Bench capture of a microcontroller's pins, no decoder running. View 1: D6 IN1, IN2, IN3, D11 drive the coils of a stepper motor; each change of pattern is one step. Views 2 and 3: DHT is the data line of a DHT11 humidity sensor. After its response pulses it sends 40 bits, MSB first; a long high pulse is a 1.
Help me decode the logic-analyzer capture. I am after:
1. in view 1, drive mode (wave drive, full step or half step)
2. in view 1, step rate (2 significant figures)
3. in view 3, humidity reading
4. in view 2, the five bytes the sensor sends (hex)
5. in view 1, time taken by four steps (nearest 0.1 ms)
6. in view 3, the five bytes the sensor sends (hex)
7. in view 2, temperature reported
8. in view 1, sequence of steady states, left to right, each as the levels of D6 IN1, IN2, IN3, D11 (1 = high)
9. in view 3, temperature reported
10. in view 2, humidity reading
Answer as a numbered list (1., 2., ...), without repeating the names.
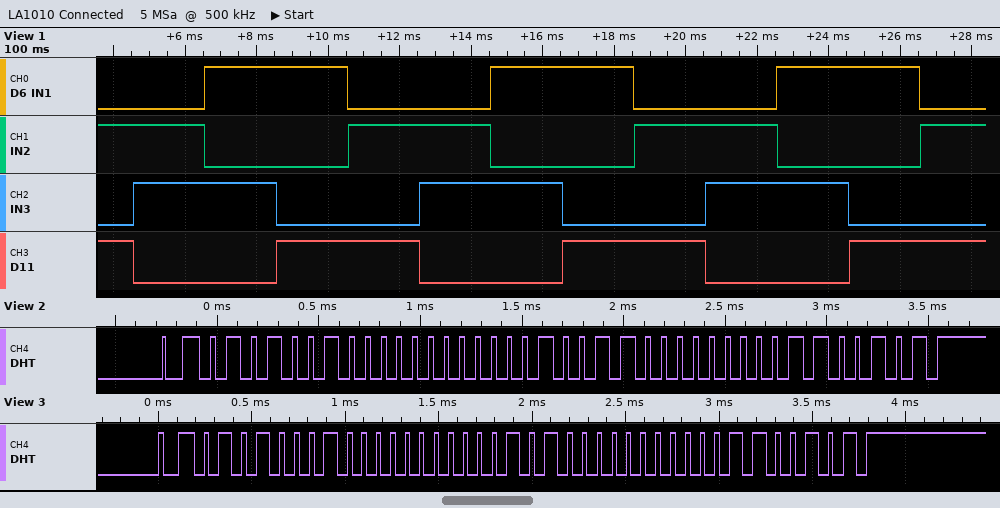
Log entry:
1. full step
2. 500 steps/s
3. 81 %
4. 52 00 13 00 65
5. 8.0 ms
6. 51 00 14 00 65
7. 19.0 °C
8. 0101 0110 1010 1001 0101 0110 1010 1001 0101 0110 1010 1001 0101
9. 20.0 °C
10. 82 %
